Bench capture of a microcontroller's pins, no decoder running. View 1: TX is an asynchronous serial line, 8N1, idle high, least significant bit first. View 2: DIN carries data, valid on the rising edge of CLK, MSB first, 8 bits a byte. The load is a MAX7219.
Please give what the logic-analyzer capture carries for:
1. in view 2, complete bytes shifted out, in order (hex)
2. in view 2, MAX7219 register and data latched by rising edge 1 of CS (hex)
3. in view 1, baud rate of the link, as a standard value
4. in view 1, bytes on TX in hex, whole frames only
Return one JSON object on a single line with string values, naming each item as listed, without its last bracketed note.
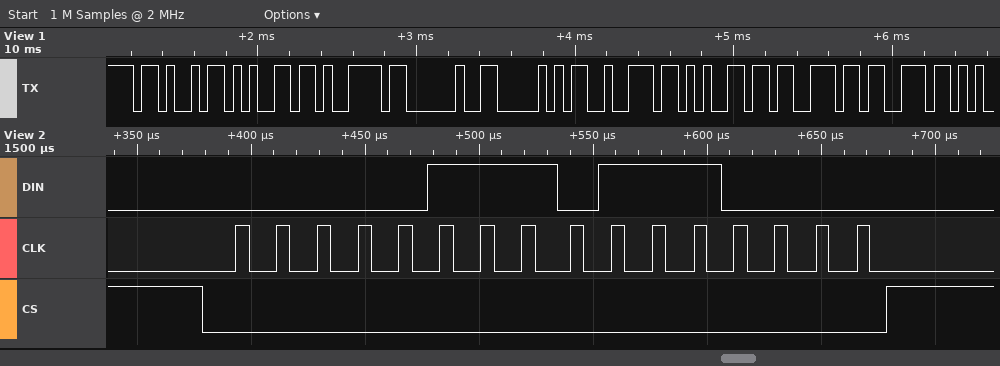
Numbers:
{"in view 2, complete bytes shifted out, in order": "07 70", "in view 2, MAX7219 register and data latched by rising edge 1 of CS": "register 0x7, data 0x70", "in view 1, baud rate of the link, as a standard value": "19200 baud", "in view 1, bytes on TX in hex, whole frames only": "4B 65 79 20 50 72 65 73 73"}
